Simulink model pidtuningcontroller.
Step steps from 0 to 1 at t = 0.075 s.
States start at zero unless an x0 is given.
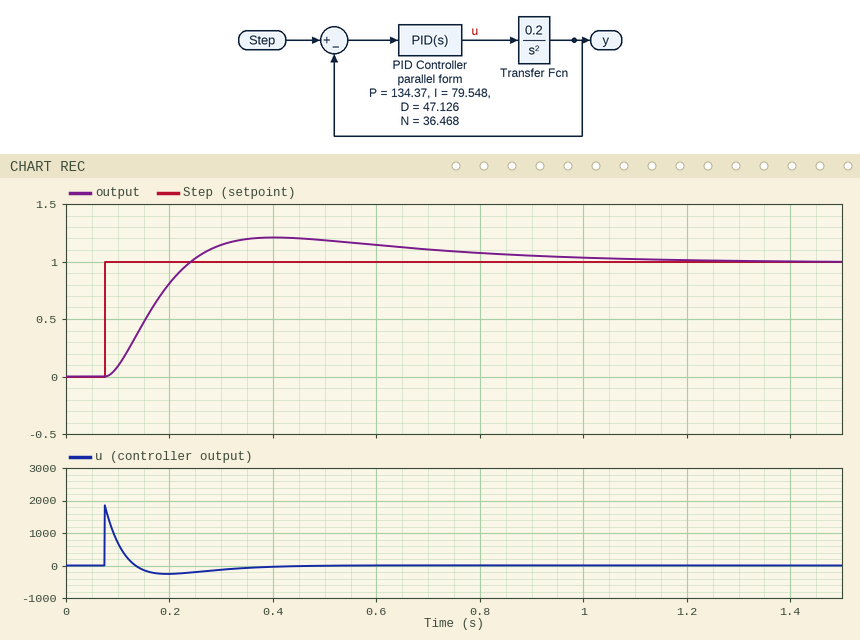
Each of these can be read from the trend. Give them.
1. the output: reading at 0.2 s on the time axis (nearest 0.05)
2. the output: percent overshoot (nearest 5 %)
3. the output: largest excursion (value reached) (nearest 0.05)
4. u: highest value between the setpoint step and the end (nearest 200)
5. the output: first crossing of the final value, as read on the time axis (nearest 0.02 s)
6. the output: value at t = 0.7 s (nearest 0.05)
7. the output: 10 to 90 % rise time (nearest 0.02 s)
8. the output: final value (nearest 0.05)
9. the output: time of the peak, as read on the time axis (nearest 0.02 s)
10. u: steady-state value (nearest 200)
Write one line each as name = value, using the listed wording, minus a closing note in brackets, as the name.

the output: reading at 0.2 s on the time axis = 0.80
the output: percent overshoot = 20 %
the output: largest excursion (value reached) = 1.20
u: highest value between the setpoint step and the end = 1800
the output: first crossing of the final value, as read on the time axis = 0.24 s
the output: value at t = 0.7 s = 1.10
the output: 10 to 90 % rise time = 0.12 s
the output: final value = 1.00
the output: time of the peak, as read on the time axis = 0.40 s
u: steady-state value = 0
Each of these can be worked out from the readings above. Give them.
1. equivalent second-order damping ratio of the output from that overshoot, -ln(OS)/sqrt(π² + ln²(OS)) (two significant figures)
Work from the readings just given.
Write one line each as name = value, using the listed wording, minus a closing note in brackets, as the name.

equivalent second-order damping ratio of the output from that overshoot, -ln(OS)/sqrt(π² + ln²(OS)) = 0.46
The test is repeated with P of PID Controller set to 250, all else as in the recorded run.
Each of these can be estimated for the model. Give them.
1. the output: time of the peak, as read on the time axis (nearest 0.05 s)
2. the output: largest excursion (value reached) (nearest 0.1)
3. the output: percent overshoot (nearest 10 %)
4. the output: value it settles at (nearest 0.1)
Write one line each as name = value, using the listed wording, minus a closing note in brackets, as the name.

the output: time of the peak, as read on the time axis = 0.35 s
the output: largest excursion (value reached) = 1.3
the output: percent overshoot = 30 %
the output: value it settles at = 1.0
